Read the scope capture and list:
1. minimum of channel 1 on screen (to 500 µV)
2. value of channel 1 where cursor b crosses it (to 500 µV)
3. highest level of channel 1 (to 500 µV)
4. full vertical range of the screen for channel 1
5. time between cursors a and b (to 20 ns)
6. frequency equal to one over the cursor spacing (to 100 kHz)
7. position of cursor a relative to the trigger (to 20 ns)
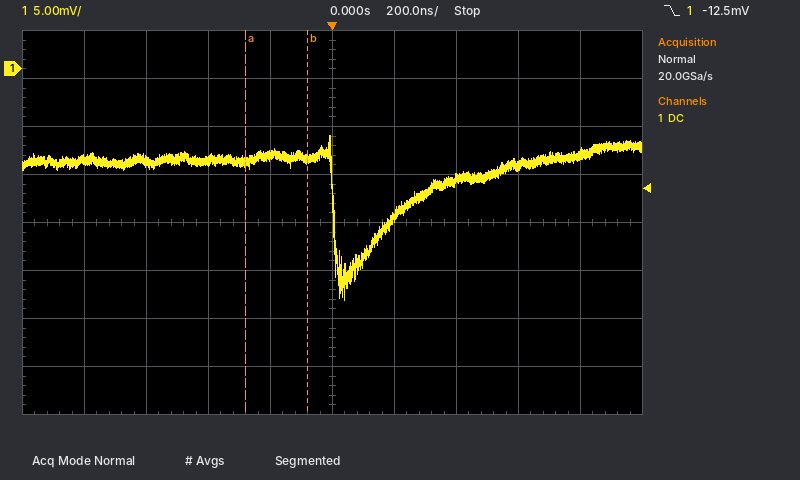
-24.0 mV
-9.5 mV
-7.0 mV
40 mV
200 ns
5.0 MHz
-280 ns
